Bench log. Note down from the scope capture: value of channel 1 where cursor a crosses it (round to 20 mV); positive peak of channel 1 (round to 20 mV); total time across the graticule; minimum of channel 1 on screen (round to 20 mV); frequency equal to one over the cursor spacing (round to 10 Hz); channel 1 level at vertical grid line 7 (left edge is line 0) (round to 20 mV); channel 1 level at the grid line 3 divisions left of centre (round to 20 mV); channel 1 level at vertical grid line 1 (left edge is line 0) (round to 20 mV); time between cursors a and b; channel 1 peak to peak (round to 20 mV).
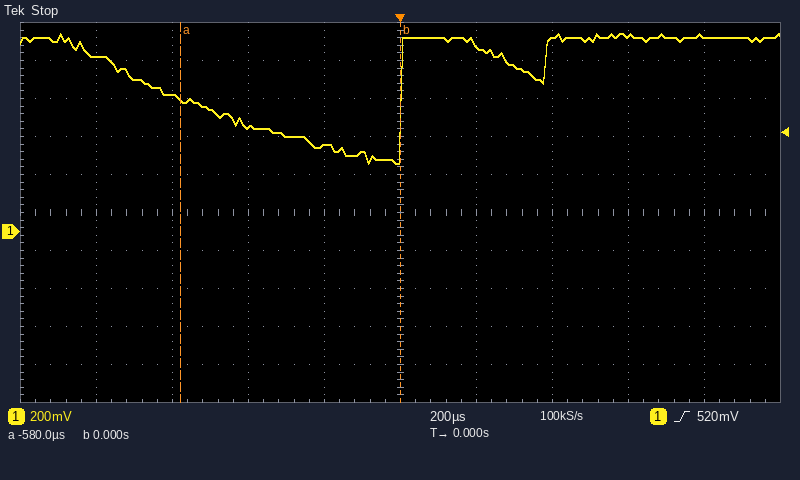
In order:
700 mV
1.04 V
2 ms
360 mV
1.72 kHz
1.02 V
720 mV
920 mV
580 µs
680 mV
